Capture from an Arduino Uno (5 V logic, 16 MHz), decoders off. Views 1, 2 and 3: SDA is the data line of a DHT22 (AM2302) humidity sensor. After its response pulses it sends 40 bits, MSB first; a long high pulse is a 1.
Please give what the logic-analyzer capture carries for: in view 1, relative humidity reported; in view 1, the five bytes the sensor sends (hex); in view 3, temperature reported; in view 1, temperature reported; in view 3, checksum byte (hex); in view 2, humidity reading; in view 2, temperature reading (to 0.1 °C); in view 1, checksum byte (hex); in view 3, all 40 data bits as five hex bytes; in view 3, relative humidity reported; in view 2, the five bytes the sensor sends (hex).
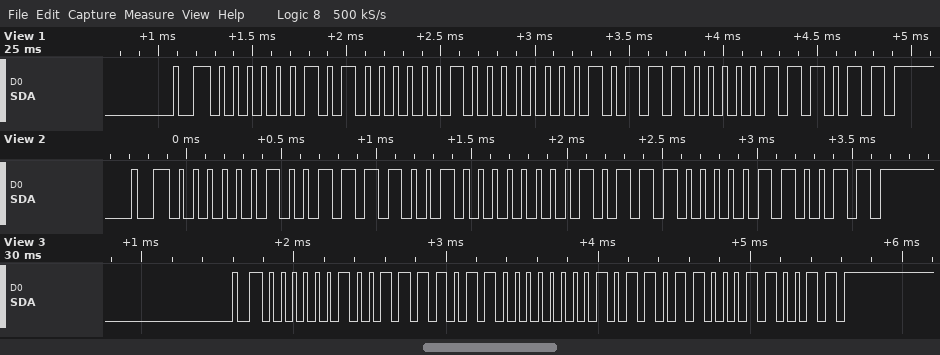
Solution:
64.1 %
02 81 00 B8 3B
18.2 °C
18.4 °C
0x33
63.3 %
18.4 °C
0x3B
02 7B 00 B6 33
63.5 %
02 79 00 B8 33
